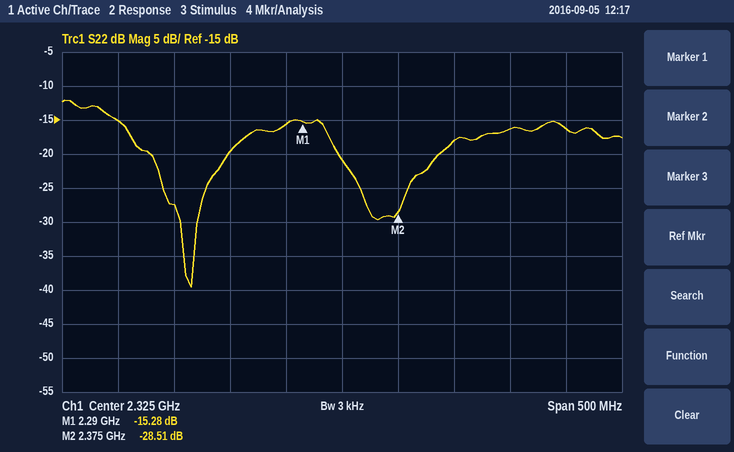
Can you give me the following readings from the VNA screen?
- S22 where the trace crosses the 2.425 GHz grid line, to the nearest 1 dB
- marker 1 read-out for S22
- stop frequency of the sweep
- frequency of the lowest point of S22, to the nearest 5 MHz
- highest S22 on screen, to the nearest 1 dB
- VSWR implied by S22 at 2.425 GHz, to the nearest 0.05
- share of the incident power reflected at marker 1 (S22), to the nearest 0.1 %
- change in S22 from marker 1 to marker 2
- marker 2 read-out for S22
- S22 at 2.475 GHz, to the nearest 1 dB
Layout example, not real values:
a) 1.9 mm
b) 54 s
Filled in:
a) -18 dB
b) -15.28 dB
c) 2.575 GHz
d) 2.190 GHz
e) -12 dB
f) 1.30
g) 3.0 %
h) -13.23 dB
i) -28.51 dB
j) -16 dB
